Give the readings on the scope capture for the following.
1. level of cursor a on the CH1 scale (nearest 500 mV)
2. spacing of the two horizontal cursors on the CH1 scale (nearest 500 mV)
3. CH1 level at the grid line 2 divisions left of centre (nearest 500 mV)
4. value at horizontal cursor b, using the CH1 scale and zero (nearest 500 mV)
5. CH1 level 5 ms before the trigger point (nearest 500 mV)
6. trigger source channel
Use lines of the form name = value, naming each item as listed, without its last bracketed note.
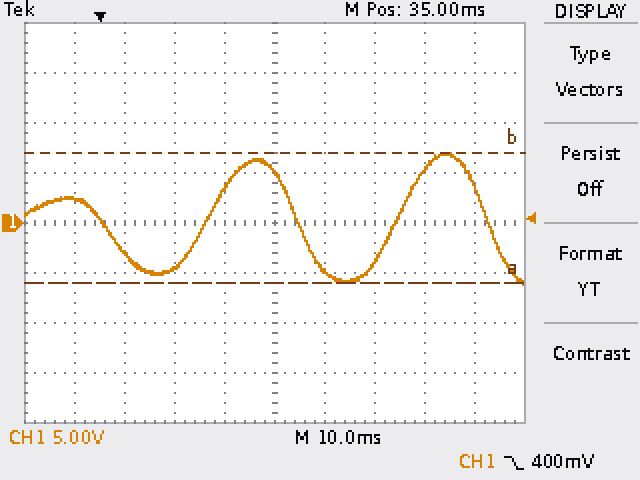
level of cursor a on the CH1 scale = -6.0 V
spacing of the two horizontal cursors on the CH1 scale = 13.0 V
CH1 level at the grid line 2 divisions left of centre = -4.5 V
value at horizontal cursor b, using the CH1 scale and zero = 7.0 V
CH1 level 5 ms before the trigger point = 2.5 V
trigger source channel = CH1
